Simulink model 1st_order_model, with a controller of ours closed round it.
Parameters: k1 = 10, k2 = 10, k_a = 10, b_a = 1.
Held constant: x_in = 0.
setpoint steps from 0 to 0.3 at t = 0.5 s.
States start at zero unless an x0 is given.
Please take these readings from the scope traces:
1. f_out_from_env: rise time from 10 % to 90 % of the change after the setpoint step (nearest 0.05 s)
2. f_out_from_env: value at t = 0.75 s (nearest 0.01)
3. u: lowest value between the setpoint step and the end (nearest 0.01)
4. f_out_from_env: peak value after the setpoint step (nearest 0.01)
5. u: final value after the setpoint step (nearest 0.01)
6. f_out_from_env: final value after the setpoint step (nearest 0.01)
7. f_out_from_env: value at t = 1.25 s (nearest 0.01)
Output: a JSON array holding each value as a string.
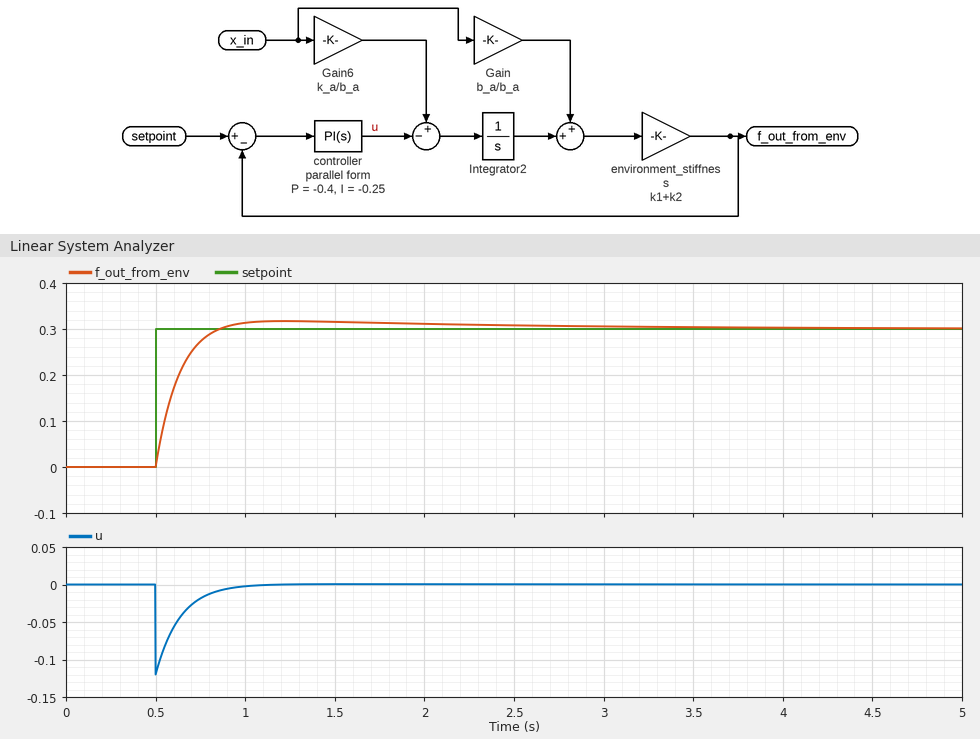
["0.25 s", "0.27", "-0.12", "0.32", "0.00", "0.30", "0.32"]
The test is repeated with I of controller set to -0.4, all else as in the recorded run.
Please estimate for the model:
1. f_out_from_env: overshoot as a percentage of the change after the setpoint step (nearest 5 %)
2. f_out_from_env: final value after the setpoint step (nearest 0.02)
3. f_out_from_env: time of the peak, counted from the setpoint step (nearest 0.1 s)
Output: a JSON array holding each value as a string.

["10 %", "0.30", "0.6 s"]
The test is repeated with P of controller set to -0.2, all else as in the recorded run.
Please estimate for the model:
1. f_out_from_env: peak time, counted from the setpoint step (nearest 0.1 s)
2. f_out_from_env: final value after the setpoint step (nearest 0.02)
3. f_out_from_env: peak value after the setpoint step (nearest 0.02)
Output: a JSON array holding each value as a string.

["0.9 s", "0.30", "0.34"]
